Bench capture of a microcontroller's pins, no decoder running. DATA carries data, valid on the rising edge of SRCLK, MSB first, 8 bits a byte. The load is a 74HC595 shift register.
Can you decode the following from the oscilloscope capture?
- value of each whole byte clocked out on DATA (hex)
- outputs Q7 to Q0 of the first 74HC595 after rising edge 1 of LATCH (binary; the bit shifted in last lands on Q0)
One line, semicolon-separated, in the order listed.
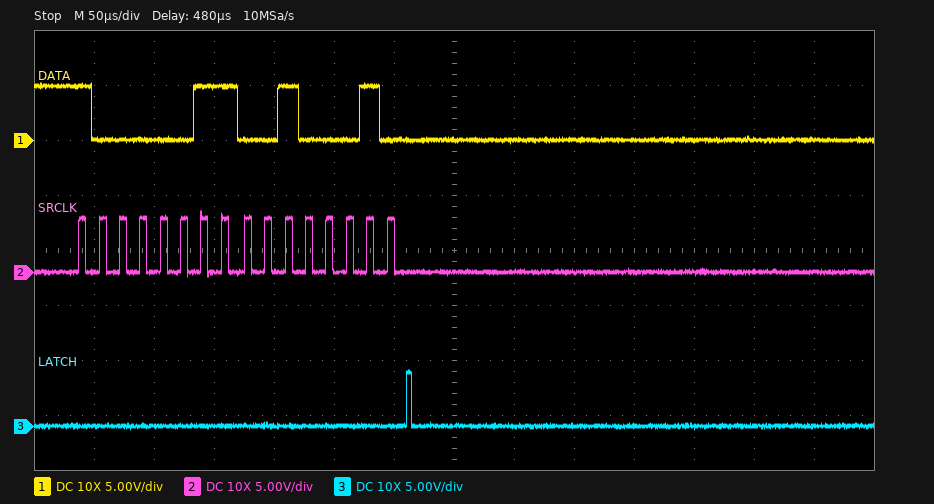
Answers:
0x83 0x22; 00100010
